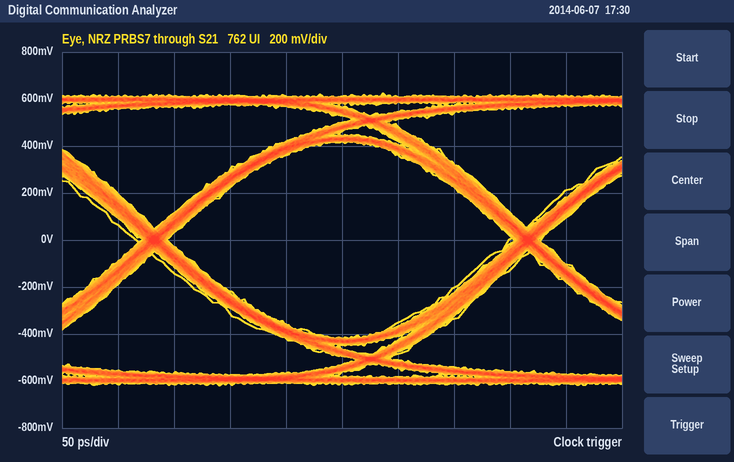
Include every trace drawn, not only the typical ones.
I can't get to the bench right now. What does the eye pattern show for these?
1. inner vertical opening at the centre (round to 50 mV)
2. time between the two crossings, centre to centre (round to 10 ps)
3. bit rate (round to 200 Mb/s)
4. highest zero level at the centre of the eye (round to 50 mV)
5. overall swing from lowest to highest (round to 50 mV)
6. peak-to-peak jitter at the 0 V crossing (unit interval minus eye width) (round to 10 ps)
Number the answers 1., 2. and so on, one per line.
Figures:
1. 850 mV
2. 330 ps
3. 3.0 Gb/s
4. -400 mV
5. 1.25 V
6. 30 ps
